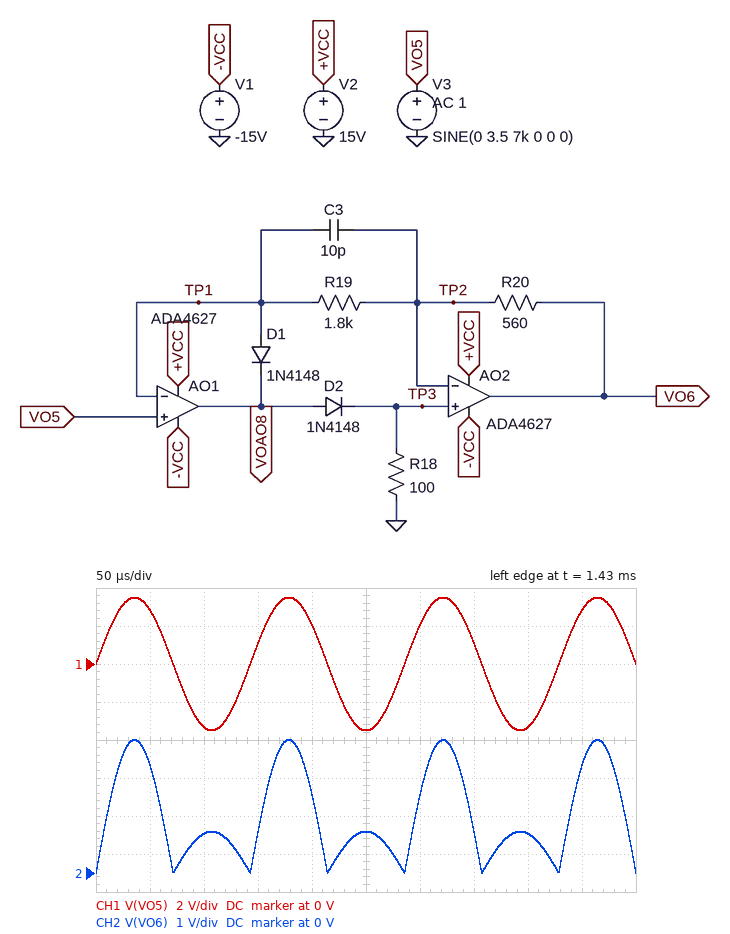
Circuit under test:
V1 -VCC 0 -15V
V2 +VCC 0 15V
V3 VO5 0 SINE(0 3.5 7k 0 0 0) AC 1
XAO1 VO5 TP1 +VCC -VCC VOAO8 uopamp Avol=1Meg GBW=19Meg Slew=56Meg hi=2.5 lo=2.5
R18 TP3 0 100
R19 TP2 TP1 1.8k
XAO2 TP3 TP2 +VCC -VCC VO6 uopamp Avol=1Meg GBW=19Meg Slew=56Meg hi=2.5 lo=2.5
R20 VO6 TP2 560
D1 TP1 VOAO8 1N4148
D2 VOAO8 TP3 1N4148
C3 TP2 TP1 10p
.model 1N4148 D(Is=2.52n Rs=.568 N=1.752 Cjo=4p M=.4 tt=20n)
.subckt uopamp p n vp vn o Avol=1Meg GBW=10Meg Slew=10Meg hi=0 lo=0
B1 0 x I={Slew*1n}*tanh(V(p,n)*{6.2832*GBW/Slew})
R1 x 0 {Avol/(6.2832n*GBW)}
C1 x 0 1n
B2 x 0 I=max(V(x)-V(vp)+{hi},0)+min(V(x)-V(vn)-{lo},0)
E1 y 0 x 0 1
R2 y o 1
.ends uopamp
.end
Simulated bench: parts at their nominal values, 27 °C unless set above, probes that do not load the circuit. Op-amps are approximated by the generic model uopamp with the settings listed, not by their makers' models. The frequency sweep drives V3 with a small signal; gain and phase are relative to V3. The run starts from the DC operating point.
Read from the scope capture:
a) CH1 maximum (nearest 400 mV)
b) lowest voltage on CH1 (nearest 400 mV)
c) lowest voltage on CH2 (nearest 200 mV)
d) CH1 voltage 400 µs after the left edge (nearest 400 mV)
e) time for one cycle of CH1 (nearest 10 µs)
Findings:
3.6 V
-3.6 V
0 V
-3.2 V
140 µs
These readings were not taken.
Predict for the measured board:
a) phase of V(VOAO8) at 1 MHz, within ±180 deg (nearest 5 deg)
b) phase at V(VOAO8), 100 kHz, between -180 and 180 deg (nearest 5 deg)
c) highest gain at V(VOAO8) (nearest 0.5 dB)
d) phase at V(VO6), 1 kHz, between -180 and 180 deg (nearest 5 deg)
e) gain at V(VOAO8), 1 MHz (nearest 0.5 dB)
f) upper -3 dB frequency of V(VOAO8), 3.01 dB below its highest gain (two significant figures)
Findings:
-85 deg
-90 deg
79.5 dB
160 deg
20.0 dB
1.1 kHz
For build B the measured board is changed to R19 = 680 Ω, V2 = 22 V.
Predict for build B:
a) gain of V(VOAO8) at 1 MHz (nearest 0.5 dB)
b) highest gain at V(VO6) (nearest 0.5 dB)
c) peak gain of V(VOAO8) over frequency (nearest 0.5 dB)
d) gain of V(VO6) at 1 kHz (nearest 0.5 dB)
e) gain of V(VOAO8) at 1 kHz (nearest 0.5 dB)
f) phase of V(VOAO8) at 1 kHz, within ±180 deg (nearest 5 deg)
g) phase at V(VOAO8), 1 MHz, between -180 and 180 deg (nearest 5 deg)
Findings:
23.0 dB
-5.0 dB
87.0 dB
-9.5 dB
81.5 dB
-60 deg
-90 deg
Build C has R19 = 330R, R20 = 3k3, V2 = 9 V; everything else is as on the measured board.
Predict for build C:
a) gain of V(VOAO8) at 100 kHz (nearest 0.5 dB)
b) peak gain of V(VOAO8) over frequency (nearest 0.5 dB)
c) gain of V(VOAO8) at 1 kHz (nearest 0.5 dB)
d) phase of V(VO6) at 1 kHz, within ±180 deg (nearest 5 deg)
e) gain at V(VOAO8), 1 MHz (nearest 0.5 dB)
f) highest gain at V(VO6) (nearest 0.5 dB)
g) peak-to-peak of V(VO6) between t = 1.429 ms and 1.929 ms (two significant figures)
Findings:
44.0 dB
92.0 dB
83.5 dB
135 deg
24.0 dB
17.0 dB
6.6 V
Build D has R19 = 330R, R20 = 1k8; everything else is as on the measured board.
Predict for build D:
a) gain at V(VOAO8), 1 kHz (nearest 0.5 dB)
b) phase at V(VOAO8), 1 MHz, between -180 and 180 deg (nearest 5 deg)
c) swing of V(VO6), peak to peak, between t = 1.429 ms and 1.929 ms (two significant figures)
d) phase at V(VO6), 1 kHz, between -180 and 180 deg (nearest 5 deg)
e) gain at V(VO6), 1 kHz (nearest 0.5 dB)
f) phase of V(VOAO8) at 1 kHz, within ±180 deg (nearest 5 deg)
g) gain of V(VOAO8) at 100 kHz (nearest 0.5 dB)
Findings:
83.5 dB
-90 deg
13 V
135 deg
3.5 dB
-70 deg
44.0 dB
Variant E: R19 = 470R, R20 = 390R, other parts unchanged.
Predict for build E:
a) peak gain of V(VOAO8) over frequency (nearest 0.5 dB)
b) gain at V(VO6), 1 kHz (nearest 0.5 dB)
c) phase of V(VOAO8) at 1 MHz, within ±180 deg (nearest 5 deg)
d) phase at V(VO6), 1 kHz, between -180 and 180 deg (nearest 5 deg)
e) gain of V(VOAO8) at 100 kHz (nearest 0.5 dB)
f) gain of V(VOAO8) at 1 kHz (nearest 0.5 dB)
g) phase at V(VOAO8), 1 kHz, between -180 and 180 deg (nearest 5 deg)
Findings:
89.5 dB
-12.5 dB
-90 deg
140 deg
43.5 dB
82.5 dB
-65 deg
